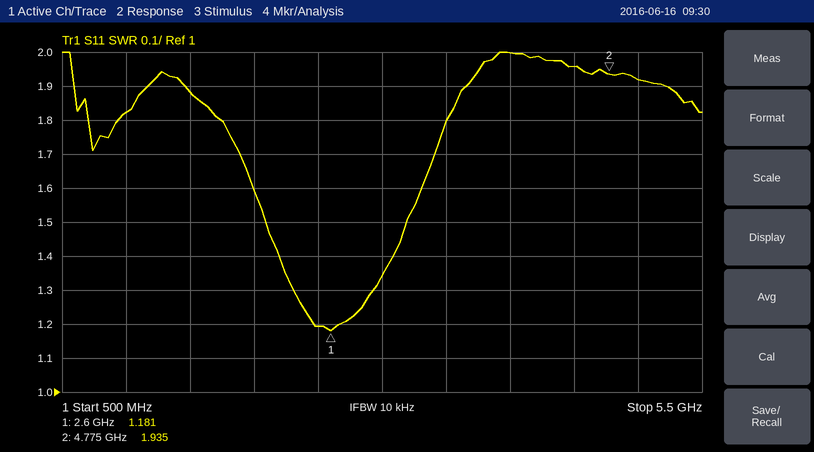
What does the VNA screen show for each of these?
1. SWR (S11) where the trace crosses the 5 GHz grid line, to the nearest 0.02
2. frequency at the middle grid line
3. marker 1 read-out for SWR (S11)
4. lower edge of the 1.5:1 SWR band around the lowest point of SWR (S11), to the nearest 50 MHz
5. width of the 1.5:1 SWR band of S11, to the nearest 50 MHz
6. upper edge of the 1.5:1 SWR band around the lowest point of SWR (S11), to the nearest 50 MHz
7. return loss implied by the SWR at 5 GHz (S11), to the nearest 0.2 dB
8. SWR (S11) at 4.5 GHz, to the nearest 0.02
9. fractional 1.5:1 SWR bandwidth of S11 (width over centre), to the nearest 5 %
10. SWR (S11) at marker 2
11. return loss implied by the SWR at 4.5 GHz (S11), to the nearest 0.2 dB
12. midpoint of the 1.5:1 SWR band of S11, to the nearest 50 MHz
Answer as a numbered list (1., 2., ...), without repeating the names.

1. 1.92
2. 3 GHz
3. 1.181
4. 2.10 GHz
5. 1.10 GHz
6. 3.20 GHz
7. 10.0 dB
8. 1.96
9. 40 %
10. 1.935
11. 9.8 dB
12. 2.65 GHz
